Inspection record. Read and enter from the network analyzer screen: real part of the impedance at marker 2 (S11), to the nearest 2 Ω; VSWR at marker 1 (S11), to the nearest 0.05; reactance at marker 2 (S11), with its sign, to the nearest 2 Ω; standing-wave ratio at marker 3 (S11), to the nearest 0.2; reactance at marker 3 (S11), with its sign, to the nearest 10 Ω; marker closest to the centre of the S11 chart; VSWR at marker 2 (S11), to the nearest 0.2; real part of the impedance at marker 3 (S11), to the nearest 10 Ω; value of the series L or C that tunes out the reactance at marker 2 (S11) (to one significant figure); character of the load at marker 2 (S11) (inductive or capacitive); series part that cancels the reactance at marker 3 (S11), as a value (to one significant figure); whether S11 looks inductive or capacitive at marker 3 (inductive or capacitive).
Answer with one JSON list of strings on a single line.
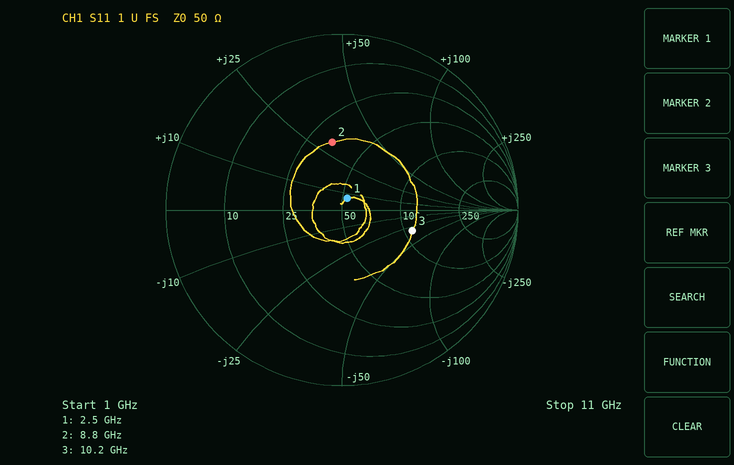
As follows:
["34 Ω", "1.15", "+30 Ω", "2.4", "-30 Ω", "marker 1", "2.2", "110 Ω", "600 fF", "inductive", "500 pH", "capacitive"]
